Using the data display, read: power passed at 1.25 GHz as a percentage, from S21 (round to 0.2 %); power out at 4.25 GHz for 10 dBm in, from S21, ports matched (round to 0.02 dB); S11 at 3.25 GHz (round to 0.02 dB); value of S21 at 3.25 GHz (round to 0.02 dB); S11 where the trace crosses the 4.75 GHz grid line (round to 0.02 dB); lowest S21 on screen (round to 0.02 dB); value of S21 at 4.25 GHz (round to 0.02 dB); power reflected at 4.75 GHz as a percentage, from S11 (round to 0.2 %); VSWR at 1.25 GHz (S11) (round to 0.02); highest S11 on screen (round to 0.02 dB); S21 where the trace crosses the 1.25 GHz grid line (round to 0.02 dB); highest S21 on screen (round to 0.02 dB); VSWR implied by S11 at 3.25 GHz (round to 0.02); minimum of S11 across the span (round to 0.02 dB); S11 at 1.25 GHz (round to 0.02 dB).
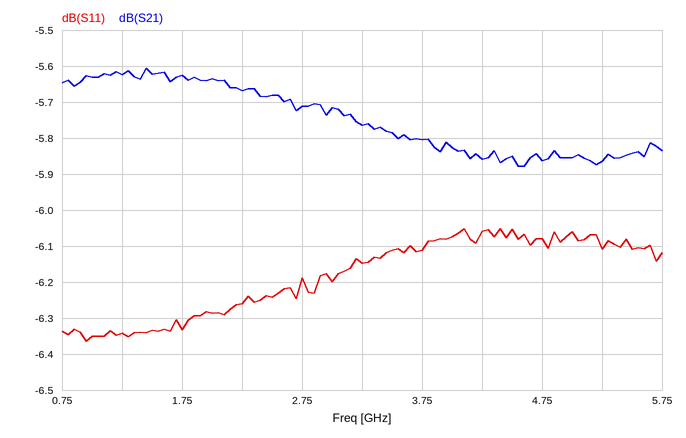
27.4 %
4.14 dBm
-6.14 dB
-5.76 dB
-6.08 dB
-5.88 dB
-5.86 dB
24.6 %
2.86
-6.06 dB
-5.62 dB
-5.60 dB
2.94
-6.36 dB
-6.34 dB
